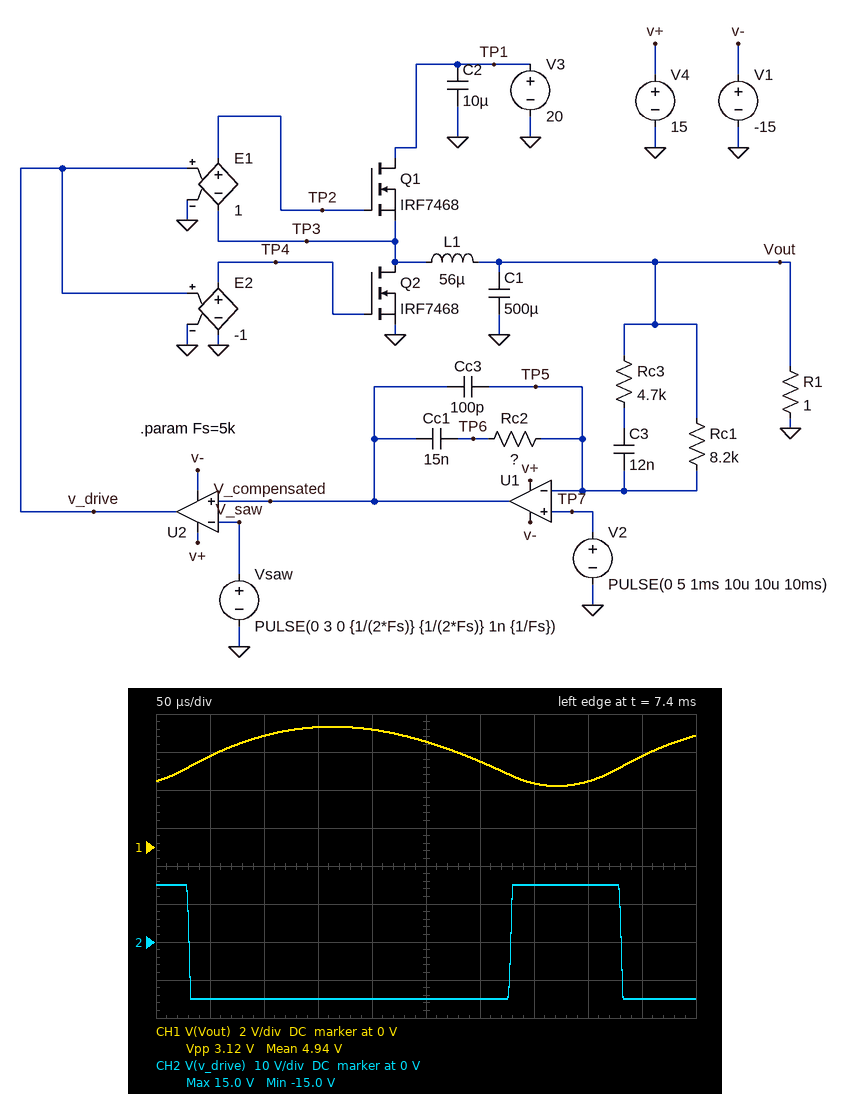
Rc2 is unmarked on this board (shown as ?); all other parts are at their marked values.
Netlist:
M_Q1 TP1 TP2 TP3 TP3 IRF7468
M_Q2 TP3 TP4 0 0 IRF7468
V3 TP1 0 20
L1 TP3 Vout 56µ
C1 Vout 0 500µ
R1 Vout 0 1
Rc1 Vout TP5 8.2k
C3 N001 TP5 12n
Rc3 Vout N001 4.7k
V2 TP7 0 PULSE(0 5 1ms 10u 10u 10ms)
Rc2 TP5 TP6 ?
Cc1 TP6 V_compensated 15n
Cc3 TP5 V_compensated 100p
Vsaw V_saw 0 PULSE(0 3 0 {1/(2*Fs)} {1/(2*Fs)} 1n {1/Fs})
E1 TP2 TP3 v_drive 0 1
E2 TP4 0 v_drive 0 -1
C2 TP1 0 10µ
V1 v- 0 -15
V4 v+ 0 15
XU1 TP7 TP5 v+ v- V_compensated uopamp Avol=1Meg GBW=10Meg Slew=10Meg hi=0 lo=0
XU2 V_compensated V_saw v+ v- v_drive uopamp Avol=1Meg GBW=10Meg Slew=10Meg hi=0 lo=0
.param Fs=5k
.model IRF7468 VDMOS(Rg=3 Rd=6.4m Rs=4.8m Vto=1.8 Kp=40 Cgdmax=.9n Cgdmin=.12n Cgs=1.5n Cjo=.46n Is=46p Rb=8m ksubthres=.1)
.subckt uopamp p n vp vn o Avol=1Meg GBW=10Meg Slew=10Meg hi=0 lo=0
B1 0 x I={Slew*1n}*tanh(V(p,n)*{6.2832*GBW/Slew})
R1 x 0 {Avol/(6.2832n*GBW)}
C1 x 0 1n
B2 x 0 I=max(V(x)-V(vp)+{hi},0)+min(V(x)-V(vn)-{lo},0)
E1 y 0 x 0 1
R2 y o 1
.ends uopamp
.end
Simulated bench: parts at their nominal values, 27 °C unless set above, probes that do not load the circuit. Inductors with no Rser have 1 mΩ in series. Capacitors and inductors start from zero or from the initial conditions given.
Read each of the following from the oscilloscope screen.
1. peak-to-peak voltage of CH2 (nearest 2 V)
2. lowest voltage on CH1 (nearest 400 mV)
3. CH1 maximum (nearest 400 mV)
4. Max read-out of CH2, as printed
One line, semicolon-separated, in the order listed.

30 V; 3.2 V; 6.4 V; 15.0 V
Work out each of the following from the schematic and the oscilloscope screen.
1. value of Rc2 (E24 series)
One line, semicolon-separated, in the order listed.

11 kΩ
